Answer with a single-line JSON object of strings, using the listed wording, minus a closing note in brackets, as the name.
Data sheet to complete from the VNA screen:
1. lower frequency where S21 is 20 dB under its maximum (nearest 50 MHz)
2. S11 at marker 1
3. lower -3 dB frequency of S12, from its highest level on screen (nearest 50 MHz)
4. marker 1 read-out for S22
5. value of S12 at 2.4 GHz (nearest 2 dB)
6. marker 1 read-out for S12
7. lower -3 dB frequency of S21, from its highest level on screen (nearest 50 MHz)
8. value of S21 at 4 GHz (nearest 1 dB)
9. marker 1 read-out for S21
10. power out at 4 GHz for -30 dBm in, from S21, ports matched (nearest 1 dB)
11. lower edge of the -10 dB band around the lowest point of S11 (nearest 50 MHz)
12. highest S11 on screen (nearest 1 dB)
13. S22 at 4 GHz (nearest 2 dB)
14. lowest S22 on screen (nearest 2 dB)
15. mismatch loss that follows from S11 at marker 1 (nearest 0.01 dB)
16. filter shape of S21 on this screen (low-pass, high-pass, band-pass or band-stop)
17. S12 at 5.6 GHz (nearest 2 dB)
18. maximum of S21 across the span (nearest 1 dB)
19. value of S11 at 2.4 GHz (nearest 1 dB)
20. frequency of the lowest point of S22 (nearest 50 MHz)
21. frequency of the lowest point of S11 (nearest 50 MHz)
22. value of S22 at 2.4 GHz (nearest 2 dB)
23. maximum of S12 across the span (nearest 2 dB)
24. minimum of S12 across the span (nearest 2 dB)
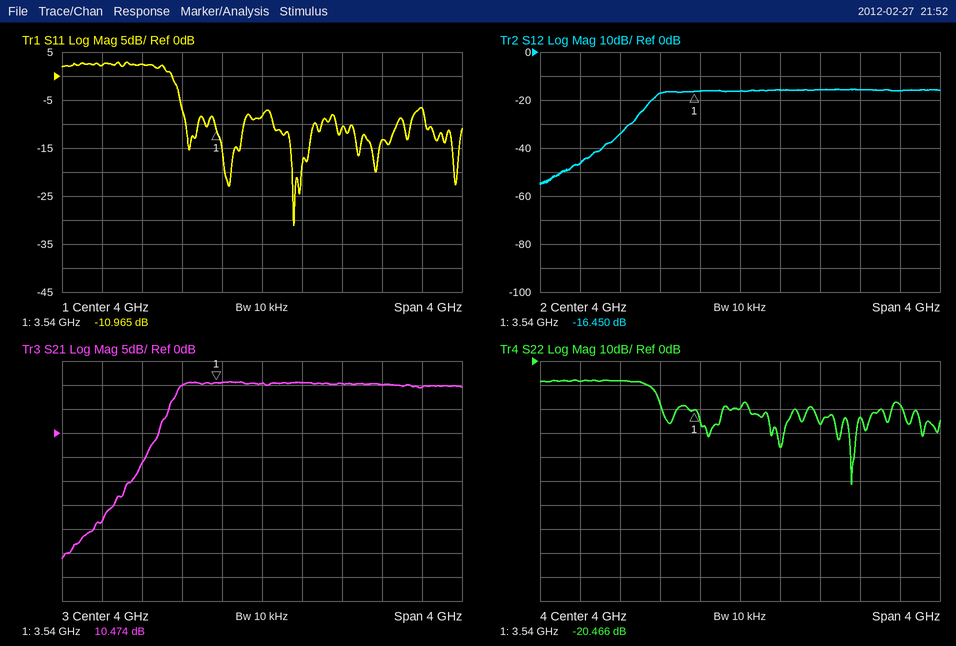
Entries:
{"lower frequency where S21 is 20 dB under its maximum": "2.70 GHz", "S11 at marker 1": "-10.965 dB", "lower -3 dB frequency of S12, from its highest level on screen": "3.15 GHz", "marker 1 read-out for S22": "-20.466 dB", "value of S12 at 2.4 GHz": "-46 dB", "marker 1 read-out for S12": "-16.450 dB", "lower -3 dB frequency of S21, from its highest level on screen": "3.15 GHz", "value of S21 at 4 GHz": "10 dB", "marker 1 read-out for S21": "10.474 dB", "power out at 4 GHz for -30 dBm in, from S21, ports matched": "-20 dBm", "lower edge of the -10 dB band around the lowest point of S11": "4.10 GHz", "highest S11 on screen": "3 dB", "S22 at 4 GHz": "-20 dB", "lowest S22 on screen": "-52 dB", "mismatch loss that follows from S11 at marker 1": "0.36 dB", "filter shape of S21 on this screen": "high-pass", "S12 at 5.6 GHz": "-16 dB", "maximum of S21 across the span": "11 dB", "value of S11 at 2.4 GHz": "2 dB", "frequency of the lowest point of S22": "5.10 GHz", "frequency of the lowest point of S11": "4.30 GHz", "value of S22 at 2.4 GHz": "-8 dB", "maximum of S12 across the span": "-16 dB", "minimum of S12 across the span": "-56 dB"}
